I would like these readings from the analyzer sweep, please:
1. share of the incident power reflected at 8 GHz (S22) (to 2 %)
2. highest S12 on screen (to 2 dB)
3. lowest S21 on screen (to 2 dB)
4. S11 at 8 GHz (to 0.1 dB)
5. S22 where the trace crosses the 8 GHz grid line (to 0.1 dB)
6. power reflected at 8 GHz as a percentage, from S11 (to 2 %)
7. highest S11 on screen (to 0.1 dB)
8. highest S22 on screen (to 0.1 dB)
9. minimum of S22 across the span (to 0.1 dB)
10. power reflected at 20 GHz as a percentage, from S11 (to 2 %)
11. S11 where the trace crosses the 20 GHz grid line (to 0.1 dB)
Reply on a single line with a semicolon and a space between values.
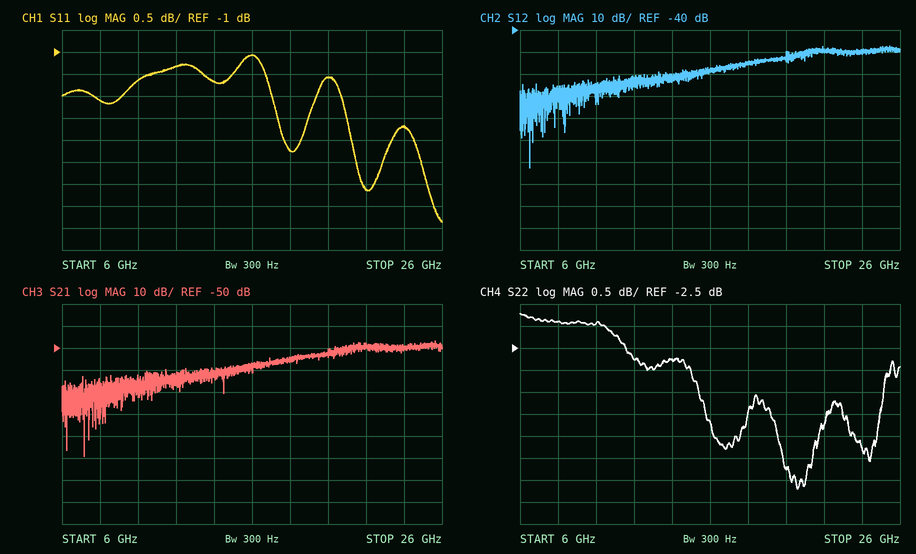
64 %; -48 dB; -100 dB; -2.1 dB; -1.9 dB; 62 %; -1.1 dB; -1.7 dB; -5.7 dB; 70 %; -1.6 dB
